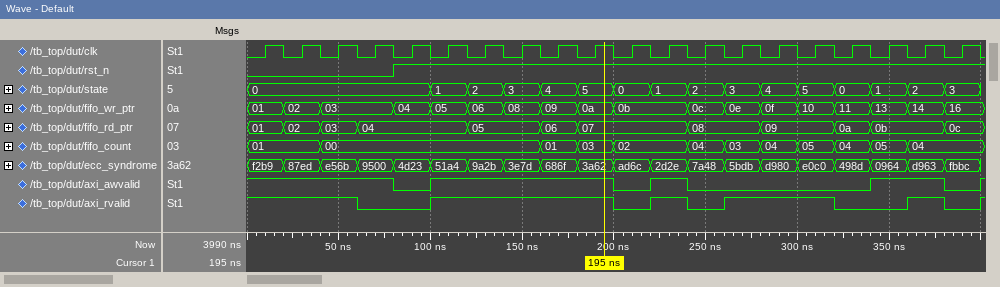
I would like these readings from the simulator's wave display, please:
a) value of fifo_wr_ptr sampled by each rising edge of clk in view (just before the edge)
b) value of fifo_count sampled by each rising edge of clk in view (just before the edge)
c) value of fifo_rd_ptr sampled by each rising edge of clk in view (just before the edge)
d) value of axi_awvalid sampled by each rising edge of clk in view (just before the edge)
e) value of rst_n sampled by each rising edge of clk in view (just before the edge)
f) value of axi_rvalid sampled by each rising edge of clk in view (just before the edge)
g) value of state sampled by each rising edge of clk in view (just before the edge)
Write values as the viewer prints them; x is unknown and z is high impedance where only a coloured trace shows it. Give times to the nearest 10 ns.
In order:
01, 02, 03, 03, 04, 05, 06, 08, 09, 0a, 0b, 0b, 0c, 0e, 0f, 10, 11, 13, 14, 16
01, 01, 00, 00, 00, 00, 00, 00, 01, 03, 02, 02, 04, 03, 04, 05, 04, 05, 04, 04
01, 02, 03, 04, 04, 04, 05, 05, 06, 07, 07, 07, 08, 08, 09, 09, 0a, 0b, 0b, 0c
1 1 1 1 0 1 1 1 1 1 0 1 0 0 0 0 0 1 1 0
0 0 0 0 1 1 1 1 1 1 1 1 1 1 1 1 1 1 1 1
1 1 1 0 0 1 1 1 1 1 0 1 0 1 1 1 0 0 1 0
0, 0, 0, 0, 0, 1, 2, 3, 4, 5, 0, 1, 2, 3, 4, 5, 0, 1, 2, 3
